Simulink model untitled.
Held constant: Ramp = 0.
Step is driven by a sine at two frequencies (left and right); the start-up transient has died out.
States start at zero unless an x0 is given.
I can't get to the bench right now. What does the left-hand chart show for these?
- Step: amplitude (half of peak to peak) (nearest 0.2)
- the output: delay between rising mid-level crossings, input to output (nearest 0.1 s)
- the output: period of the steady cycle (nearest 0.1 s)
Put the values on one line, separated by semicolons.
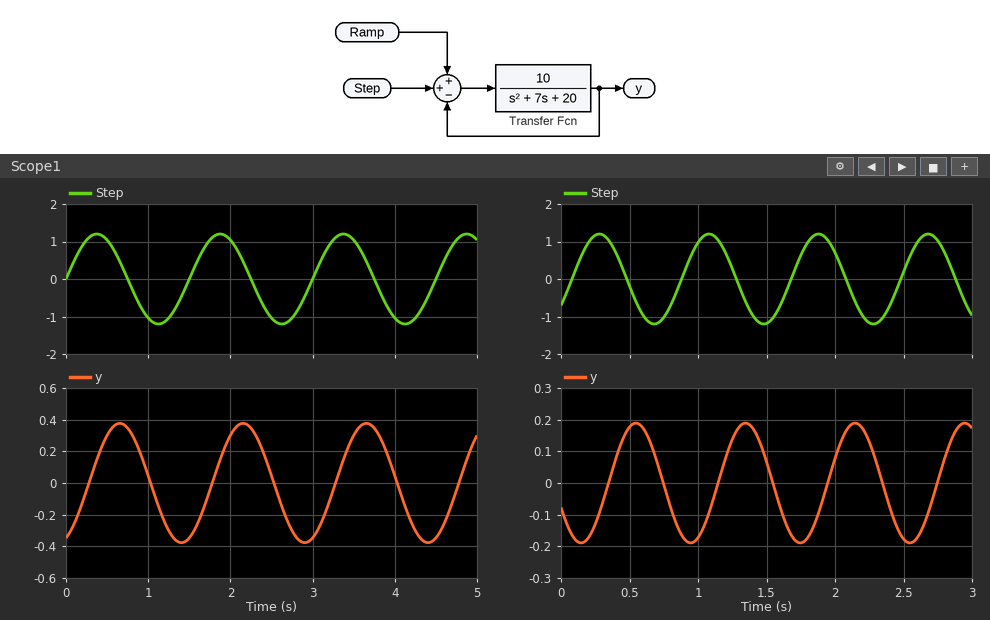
1.2; 0.3 s; 1.5 s
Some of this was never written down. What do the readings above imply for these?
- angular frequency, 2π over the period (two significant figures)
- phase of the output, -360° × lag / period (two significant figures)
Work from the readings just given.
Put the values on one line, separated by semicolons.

4.2 rad/s; -72°
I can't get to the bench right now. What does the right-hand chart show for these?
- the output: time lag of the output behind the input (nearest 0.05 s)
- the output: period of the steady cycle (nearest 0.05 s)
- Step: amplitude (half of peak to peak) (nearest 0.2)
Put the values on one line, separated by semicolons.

0.25 s; 0.80 s; 1.2
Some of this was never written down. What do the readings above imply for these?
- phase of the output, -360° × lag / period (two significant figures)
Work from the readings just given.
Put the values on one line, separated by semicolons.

-110°
